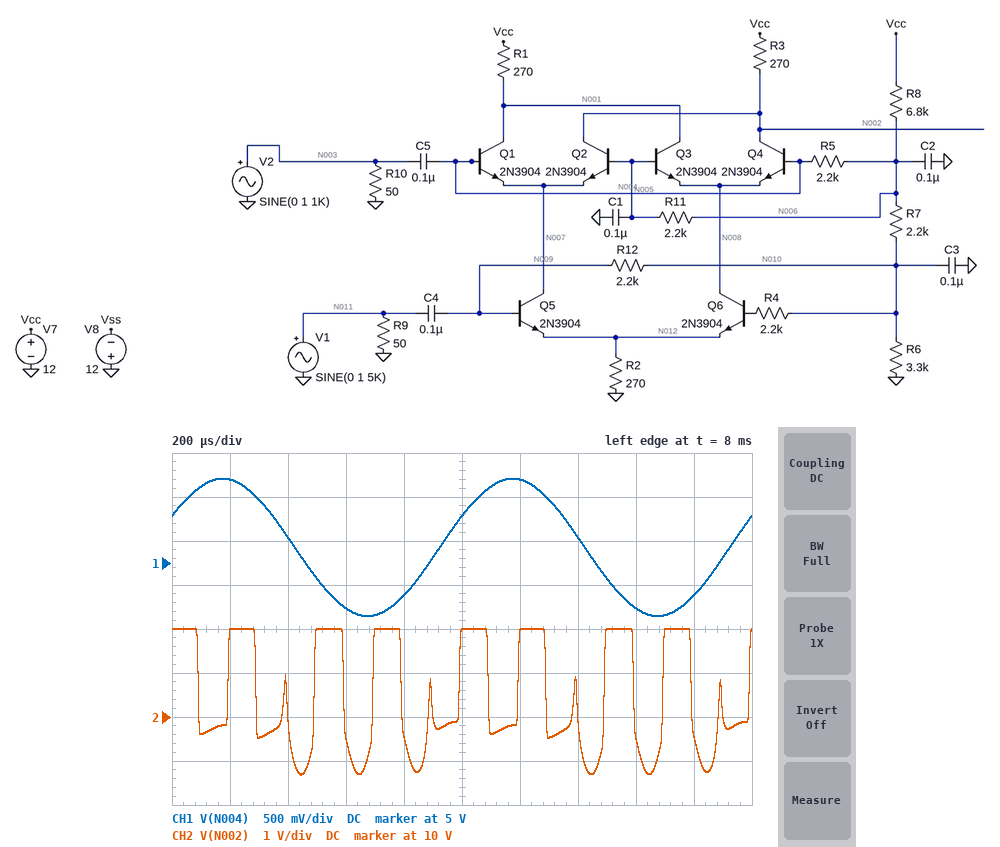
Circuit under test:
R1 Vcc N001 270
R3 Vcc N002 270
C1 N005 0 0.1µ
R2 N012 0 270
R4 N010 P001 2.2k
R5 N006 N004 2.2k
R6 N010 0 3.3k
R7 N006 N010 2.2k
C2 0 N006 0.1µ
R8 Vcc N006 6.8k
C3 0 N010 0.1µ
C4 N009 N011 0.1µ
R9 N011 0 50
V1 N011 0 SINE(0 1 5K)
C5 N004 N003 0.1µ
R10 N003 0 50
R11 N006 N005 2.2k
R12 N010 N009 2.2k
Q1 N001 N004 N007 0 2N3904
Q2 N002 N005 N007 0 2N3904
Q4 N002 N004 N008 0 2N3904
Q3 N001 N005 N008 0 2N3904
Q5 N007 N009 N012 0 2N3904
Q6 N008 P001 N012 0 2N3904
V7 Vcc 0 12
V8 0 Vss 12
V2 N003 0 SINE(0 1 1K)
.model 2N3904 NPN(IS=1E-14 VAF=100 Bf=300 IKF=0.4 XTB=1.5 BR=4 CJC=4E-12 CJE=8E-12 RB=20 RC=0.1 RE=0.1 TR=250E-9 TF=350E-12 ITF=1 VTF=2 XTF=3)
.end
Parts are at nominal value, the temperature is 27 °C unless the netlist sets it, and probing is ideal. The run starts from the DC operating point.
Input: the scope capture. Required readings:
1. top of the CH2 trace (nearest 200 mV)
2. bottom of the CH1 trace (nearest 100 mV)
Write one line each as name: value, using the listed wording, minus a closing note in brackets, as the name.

top of the CH2 trace: 12.0 V
bottom of the CH1 trace: 4.4 V
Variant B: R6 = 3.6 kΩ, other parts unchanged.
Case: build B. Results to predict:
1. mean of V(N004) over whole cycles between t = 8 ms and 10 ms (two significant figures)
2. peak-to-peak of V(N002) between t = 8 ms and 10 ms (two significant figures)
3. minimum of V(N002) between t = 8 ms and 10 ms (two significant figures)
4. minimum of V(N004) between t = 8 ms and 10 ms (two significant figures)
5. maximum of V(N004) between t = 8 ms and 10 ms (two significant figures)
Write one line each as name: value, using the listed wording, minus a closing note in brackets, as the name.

mean of V(N004) over whole cycles between t = 8 ms and 10 ms: 5.3 V
peak-to-peak of V(N002) between t = 8 ms and 10 ms: 3.5 V
minimum of V(N002) between t = 8 ms and 10 ms: 8.5 V
minimum of V(N004) between t = 8 ms and 10 ms: 4.5 V
maximum of V(N004) between t = 8 ms and 10 ms: 6.1 V
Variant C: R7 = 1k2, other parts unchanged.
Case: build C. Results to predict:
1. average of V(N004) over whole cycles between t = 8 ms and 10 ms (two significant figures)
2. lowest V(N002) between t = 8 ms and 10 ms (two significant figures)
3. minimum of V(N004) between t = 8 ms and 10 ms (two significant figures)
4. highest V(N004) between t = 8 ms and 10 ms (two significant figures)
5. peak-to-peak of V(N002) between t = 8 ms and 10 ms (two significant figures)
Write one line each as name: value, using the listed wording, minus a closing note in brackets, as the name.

average of V(N004) over whole cycles between t = 8 ms and 10 ms: 4.6 V
lowest V(N002) between t = 8 ms and 10 ms: 8.4 V
minimum of V(N004) between t = 8 ms and 10 ms: 3.8 V
highest V(N004) between t = 8 ms and 10 ms: 5.4 V
peak-to-peak of V(N002) between t = 8 ms and 10 ms: 3.6 V
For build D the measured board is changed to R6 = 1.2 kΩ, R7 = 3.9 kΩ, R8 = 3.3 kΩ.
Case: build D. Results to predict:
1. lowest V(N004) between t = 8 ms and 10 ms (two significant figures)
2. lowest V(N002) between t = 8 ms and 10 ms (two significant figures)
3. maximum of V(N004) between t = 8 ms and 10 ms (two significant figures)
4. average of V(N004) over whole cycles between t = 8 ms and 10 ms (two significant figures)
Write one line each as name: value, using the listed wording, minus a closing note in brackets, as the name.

lowest V(N004) between t = 8 ms and 10 ms: 6.4 V
lowest V(N002) between t = 8 ms and 10 ms: 10 V
maximum of V(N004) between t = 8 ms and 10 ms: 8.0 V
average of V(N004) over whole cycles between t = 8 ms and 10 ms: 7.2 V
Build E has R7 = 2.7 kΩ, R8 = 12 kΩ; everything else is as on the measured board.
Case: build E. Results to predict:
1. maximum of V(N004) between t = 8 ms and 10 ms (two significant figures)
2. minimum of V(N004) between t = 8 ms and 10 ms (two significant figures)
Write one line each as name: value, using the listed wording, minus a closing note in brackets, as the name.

maximum of V(N004) between t = 8 ms and 10 ms: 4.6 V
minimum of V(N004) between t = 8 ms and 10 ms: 3.1 V
